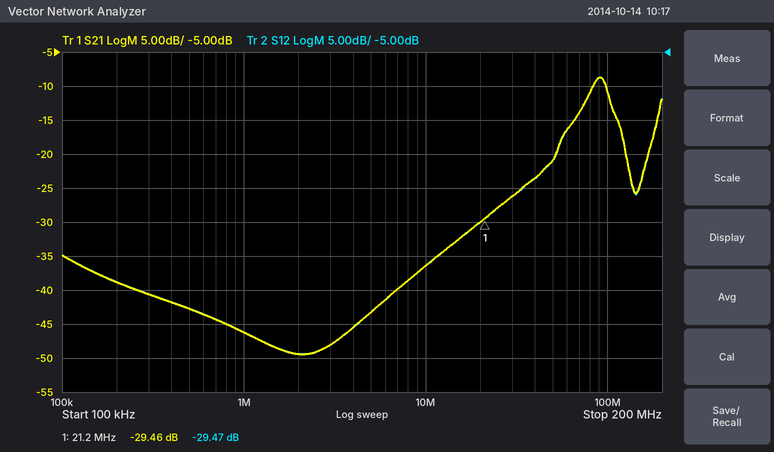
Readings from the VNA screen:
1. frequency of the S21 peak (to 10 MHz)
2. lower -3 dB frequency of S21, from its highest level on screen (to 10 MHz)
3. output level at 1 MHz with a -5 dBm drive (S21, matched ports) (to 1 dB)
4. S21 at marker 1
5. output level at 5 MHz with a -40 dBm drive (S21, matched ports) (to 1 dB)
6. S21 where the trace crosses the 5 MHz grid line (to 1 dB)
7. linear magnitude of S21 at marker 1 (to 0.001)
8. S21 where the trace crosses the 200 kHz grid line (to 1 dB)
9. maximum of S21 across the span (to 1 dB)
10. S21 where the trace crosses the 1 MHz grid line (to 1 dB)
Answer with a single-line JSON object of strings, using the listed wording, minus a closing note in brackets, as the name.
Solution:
{"frequency of the S21 peak": "90 MHz", "lower -3 dB frequency of S21, from its highest level on screen": "80 MHz", "output level at 1 MHz with a -5 dBm drive (S21, matched ports)": "-51 dBm", "S21 at marker 1": "-29.46 dB", "output level at 5 MHz with a -40 dBm drive (S21, matched ports)": "-83 dBm", "S21 where the trace crosses the 5 MHz grid line": "-43 dB", "linear magnitude of S21 at marker 1": "0.034", "S21 where the trace crosses the 200 kHz grid line": "-39 dB", "maximum of S21 across the span": "-9 dB", "S21 where the trace crosses the 1 MHz grid line": "-46 dB"}
